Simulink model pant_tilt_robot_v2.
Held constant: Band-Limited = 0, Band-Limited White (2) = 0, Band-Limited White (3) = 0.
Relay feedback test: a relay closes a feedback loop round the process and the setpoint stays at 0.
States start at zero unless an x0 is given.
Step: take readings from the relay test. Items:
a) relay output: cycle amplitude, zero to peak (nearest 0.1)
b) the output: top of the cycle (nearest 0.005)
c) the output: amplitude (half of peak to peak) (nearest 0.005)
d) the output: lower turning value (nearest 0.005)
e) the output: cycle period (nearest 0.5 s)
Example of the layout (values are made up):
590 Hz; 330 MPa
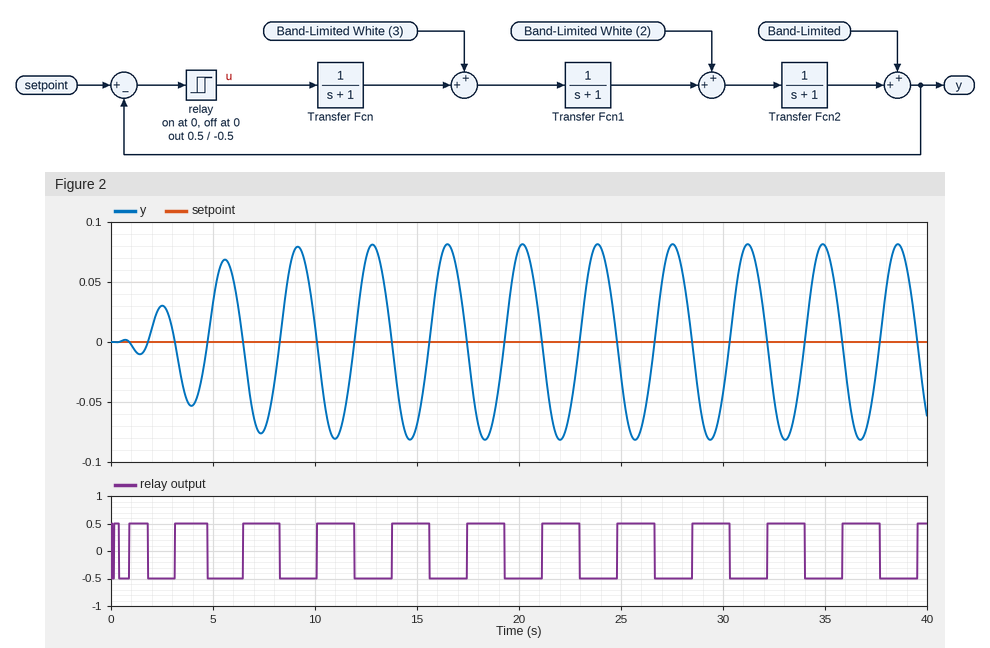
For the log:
0.5; 0.080; 0.080; -0.080; 3.5 s
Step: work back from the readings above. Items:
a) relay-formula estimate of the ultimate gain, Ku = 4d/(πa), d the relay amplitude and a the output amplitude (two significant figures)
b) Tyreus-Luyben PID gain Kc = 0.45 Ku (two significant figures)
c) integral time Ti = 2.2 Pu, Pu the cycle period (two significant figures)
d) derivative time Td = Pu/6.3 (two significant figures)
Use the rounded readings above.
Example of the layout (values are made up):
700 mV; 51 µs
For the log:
8.0; 3.6; 7.7 s; 0.56 s
